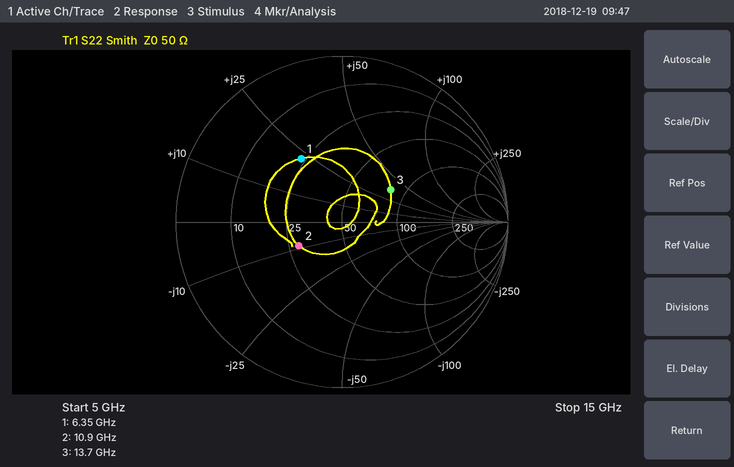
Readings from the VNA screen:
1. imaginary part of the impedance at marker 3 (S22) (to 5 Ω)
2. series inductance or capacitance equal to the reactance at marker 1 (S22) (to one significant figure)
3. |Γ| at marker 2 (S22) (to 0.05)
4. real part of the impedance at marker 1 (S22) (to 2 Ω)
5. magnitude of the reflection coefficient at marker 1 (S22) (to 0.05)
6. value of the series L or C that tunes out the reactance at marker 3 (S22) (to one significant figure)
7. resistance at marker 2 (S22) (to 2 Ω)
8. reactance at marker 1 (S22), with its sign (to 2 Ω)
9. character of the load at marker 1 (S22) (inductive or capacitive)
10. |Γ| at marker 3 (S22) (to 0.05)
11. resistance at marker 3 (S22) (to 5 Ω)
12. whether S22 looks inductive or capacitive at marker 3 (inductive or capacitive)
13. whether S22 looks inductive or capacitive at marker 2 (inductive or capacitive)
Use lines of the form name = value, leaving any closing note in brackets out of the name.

imaginary part of the impedance at marker 3 (S22) = +35 Ω
series inductance or capacitance equal to the reactance at marker 1 (S22) = 600 pH
|Γ| at marker 2 (S22) = 0.30
real part of the impedance at marker 1 (S22) = 24 Ω
magnitude of the reflection coefficient at marker 1 (S22) = 0.45
value of the series L or C that tunes out the reactance at marker 3 (S22) = 300 fF
resistance at marker 2 (S22) = 28 Ω
reactance at marker 1 (S22), with its sign = +22 Ω
character of the load at marker 1 (S22) = inductive
|Γ| at marker 3 (S22) = 0.35
resistance at marker 3 (S22) = 80 Ω
whether S22 looks inductive or capacitive at marker 3 = inductive
whether S22 looks inductive or capacitive at marker 2 = capacitive
